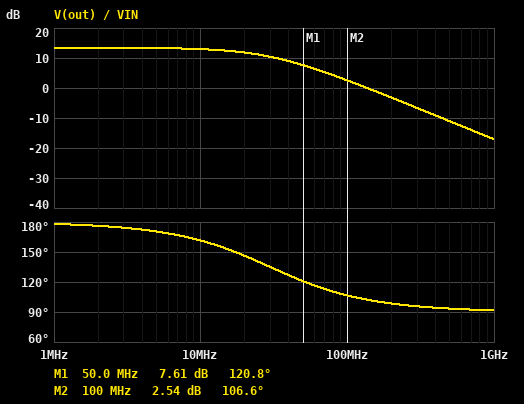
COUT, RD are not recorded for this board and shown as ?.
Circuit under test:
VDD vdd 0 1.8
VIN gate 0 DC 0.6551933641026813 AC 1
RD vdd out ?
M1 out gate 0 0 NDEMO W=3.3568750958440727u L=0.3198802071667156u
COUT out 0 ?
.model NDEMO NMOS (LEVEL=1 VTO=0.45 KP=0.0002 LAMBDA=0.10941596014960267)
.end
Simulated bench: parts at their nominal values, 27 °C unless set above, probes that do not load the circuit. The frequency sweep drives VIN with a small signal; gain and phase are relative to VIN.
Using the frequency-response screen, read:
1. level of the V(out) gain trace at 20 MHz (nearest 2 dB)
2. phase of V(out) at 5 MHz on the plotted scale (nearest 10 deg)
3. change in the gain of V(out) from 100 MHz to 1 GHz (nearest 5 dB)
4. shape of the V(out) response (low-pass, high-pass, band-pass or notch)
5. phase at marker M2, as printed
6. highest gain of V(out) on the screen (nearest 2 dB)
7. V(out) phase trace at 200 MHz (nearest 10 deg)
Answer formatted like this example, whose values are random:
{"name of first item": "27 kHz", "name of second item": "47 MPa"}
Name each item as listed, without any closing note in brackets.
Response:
{"level of the V(out) gain trace at 20 MHz": "12 dB", "phase of V(out) at 5 MHz on the plotted scale": "170 deg", "change in the gain of V(out) from 100 MHz to 1 GHz": "-20 dB", "shape of the V(out) response": "low-pass", "phase at marker M2, as printed": "106.6 deg", "highest gain of V(out) on the screen": "14 dB", "V(out) phase trace at 200 MHz": "100 deg"}
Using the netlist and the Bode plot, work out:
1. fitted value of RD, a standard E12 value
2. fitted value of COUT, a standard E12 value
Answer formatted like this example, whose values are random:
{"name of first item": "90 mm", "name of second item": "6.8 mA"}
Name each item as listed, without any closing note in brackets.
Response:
{"fitted value of RD, a standard E12 value": "10 kΩ", "fitted value of COUT, a standard E12 value": "560 fF"}
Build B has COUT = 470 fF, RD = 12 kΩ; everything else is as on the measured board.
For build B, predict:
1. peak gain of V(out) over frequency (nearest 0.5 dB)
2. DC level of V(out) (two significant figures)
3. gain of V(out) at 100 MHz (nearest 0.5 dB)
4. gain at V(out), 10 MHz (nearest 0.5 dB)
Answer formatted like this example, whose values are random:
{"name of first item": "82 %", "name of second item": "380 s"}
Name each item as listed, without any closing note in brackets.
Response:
{"peak gain of V(out) over frequency": "15.0 dB", "DC level of V(out)": "1.2 V", "gain of V(out) at 100 MHz": "4.0 dB", "gain at V(out), 10 MHz": "14.5 dB"}
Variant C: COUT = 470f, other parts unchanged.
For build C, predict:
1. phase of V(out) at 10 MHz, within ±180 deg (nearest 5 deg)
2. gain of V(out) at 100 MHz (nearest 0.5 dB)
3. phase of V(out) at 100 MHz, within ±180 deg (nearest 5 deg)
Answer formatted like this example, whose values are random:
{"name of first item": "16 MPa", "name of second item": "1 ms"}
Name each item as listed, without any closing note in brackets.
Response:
{"phase of V(out) at 10 MHz, within ±180 deg": "165 deg", "gain of V(out) at 100 MHz": "4.0 dB", "phase of V(out) at 100 MHz, within ±180 deg": "110 deg"}
